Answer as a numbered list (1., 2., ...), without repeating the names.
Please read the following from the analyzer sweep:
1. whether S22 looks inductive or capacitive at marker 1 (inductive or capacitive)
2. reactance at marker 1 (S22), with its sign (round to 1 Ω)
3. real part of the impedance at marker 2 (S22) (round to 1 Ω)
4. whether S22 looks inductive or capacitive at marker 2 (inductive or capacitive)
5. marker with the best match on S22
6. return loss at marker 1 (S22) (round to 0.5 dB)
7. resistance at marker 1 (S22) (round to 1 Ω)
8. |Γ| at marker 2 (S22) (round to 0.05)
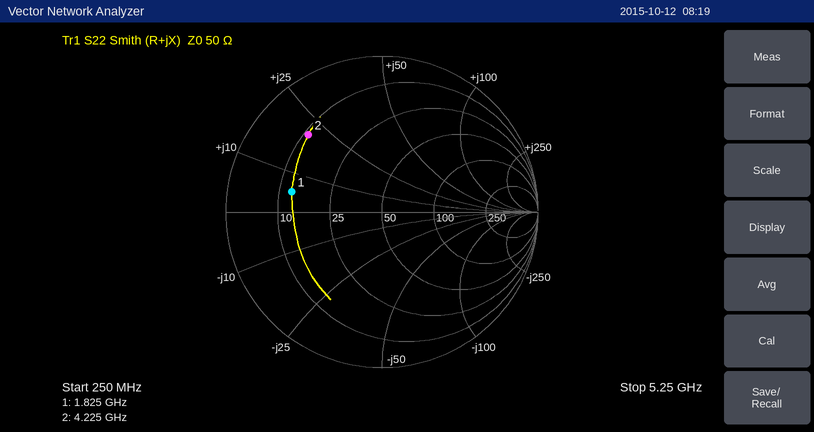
1. inductive
2. +5 Ω
3. 11 Ω
4. inductive
5. marker 1
6. 4.5 dB
7. 13 Ω
8. 0.70
